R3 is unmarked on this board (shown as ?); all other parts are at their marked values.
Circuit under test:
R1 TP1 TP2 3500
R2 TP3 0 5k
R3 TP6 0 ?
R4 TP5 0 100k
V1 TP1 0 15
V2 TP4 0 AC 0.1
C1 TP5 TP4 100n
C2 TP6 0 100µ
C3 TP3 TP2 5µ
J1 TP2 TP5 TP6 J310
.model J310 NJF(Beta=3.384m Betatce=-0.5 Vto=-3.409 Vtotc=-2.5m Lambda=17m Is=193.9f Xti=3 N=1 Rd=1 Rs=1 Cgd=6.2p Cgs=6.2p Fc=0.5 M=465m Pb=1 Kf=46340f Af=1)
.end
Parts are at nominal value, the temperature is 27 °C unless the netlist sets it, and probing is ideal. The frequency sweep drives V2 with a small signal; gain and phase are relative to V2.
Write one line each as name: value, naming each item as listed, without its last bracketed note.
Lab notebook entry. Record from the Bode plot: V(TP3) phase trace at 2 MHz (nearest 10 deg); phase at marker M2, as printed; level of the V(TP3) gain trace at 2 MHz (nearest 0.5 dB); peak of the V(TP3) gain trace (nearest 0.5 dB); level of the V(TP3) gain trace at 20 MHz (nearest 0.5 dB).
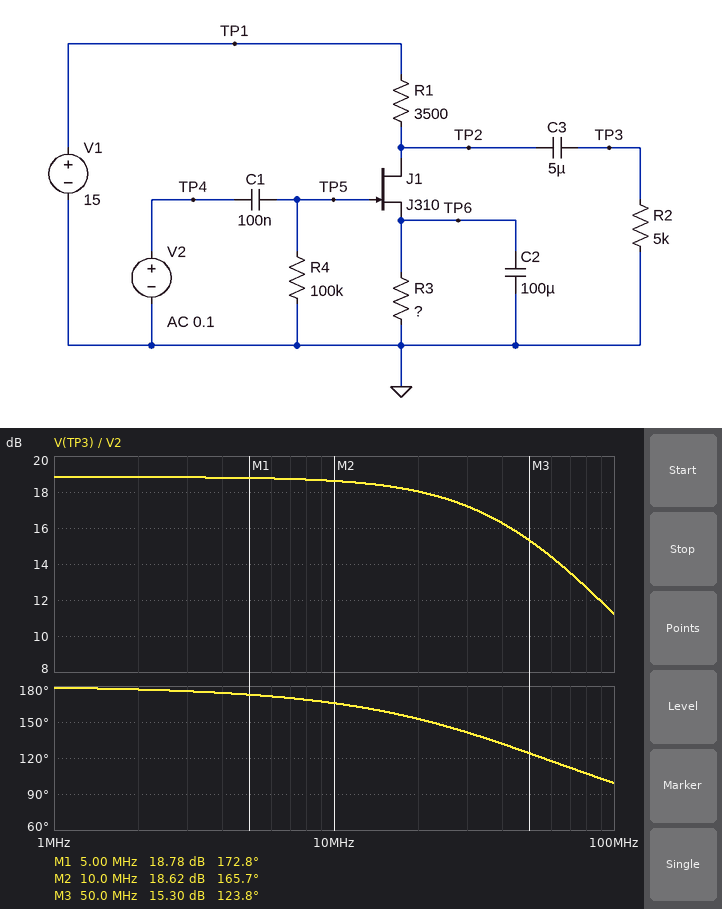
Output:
V(TP3) phase trace at 2 MHz: 180 deg
phase at marker M2, as printed: 165.7 deg
level of the V(TP3) gain trace at 2 MHz: 19.0 dB
peak of the V(TP3) gain trace: 19.0 dB
level of the V(TP3) gain trace at 20 MHz: 18.0 dB
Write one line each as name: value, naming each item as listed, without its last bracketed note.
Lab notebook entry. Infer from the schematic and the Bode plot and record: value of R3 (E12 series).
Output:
value of R3: 2.2 kΩ
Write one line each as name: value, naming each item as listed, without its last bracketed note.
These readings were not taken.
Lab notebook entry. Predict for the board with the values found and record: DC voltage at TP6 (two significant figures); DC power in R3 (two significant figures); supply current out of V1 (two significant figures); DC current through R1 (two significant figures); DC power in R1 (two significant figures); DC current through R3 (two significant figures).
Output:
DC voltage at TP6: 2.8 V
DC power in R3: 3.6 mW
supply current out of V1: 1.3 mA
DC current through R1: 1.3 mA
DC power in R1: 5.8 mW
DC current through R3: 1.3 mA
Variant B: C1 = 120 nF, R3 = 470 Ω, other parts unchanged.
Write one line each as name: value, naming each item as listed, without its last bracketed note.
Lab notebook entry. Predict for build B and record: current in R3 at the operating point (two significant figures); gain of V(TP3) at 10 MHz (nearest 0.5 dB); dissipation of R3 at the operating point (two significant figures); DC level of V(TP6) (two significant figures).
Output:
current in R3 at the operating point: 3.7 mA
gain of V(TP3) at 10 MHz: -11.5 dB
dissipation of R3 at the operating point: 6.4 mW
DC level of V(TP6): 1.7 V
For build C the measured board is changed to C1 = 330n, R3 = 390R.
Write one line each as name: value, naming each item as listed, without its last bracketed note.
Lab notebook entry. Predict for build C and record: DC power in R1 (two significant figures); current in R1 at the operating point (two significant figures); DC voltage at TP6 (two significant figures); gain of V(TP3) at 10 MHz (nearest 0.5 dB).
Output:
DC power in R1: 50 mW
current in R1 at the operating point: 3.8 mA
DC voltage at TP6: 1.5 V
gain of V(TP3) at 10 MHz: -14.5 dB
